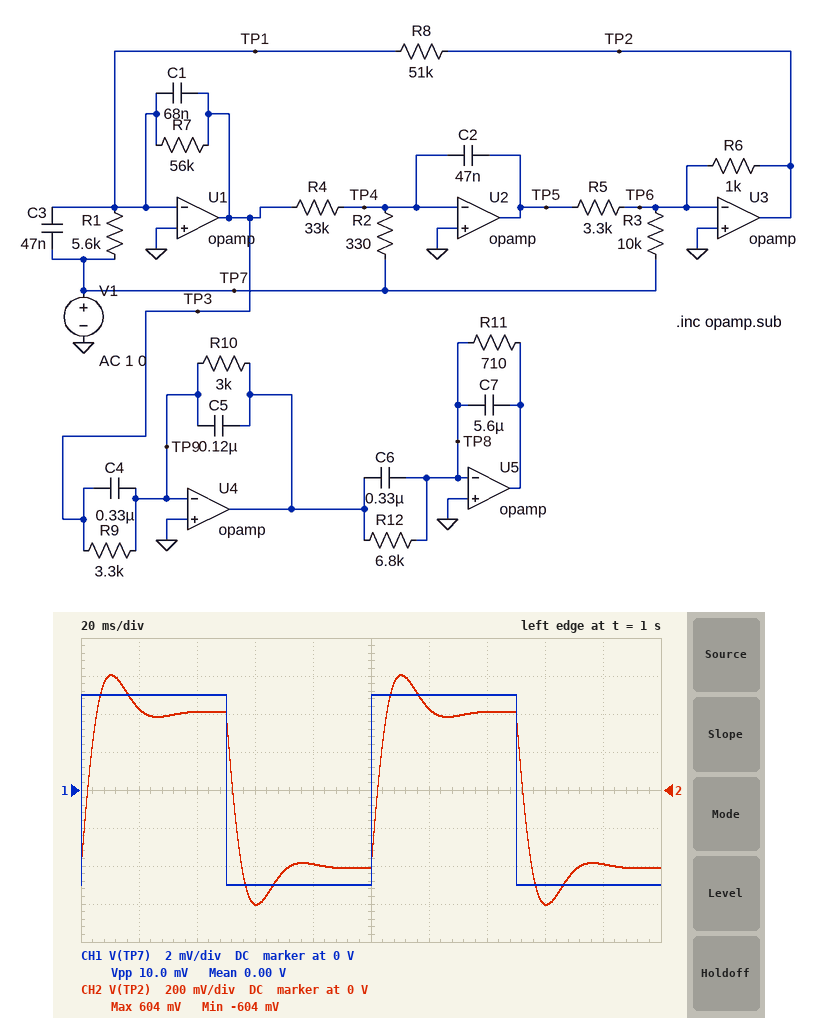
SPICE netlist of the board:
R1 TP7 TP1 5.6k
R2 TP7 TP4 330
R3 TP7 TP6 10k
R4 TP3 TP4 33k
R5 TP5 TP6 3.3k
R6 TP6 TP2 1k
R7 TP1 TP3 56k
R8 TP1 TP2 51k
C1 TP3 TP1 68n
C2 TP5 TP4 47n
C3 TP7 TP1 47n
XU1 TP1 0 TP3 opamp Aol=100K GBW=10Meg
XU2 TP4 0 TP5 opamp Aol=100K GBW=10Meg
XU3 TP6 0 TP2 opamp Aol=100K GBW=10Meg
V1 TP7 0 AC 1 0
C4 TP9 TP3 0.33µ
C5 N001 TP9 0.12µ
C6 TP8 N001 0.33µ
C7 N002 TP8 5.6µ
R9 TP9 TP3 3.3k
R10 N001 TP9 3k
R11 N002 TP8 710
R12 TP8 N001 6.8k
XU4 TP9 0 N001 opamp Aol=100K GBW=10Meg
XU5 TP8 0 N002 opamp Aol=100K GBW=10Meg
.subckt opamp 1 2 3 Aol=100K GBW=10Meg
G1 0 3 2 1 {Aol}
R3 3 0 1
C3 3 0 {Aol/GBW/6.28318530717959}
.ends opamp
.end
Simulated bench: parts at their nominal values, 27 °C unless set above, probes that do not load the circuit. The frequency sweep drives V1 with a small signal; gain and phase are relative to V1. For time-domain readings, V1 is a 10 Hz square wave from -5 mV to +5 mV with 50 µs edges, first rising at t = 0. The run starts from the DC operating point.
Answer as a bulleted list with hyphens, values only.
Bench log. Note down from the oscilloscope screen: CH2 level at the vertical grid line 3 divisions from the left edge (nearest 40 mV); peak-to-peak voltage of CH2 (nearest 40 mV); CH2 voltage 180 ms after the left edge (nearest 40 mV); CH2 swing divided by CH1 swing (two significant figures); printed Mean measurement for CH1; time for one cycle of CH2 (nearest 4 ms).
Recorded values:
- -600 mV
- 1.20 V
- -400 mV
- 120
- 0.00 V
- 100 ms
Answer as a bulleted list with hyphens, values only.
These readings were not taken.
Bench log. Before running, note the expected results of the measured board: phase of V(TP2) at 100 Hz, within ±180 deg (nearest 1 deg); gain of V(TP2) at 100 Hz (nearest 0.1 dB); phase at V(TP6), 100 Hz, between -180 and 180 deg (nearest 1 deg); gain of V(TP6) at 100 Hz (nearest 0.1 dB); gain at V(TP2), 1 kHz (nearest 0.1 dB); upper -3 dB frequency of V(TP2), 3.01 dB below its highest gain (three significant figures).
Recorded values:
- -85 deg
- 30.8 dB
- 140 deg
- -66.2 dB
- 9.8 dB
- 52.7 Hz
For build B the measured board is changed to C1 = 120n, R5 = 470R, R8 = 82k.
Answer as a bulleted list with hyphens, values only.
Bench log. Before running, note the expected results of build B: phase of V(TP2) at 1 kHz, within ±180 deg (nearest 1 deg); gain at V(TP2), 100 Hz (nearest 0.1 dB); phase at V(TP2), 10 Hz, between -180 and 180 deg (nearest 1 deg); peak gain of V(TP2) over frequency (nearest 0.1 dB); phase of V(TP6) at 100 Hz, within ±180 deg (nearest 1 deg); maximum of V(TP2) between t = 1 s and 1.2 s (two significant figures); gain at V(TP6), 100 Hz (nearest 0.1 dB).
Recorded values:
- -90 deg
- 50.2 dB
- 21 deg
- 59.7 dB
- 143 deg
- 3.2 V
- -46.8 dB
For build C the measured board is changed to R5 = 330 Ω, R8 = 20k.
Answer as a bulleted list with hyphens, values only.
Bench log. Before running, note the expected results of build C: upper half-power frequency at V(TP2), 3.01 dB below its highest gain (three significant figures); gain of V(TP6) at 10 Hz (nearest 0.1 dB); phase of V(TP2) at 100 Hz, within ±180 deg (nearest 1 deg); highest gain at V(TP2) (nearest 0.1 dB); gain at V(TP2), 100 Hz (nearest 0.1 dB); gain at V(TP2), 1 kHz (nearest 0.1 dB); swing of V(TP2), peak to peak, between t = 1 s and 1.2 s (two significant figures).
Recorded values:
- 213 Hz
- -69.5 dB
- 60 deg
- 57.5 dB
- 41.8 dB
- 30.1 dB
- 3.0 V
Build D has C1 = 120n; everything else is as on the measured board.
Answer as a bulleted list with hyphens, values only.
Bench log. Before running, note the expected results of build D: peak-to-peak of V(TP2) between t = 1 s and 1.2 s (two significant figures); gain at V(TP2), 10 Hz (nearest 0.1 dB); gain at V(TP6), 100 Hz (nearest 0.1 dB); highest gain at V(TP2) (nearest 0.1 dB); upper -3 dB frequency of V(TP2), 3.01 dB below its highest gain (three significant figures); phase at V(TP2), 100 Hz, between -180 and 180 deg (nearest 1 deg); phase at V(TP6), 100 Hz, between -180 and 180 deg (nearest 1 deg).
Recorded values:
- 1.7 V
- 39.8 dB
- -66.5 dB
- 44.3 dB
- 39.3 Hz
- -88 deg
- 137 deg
